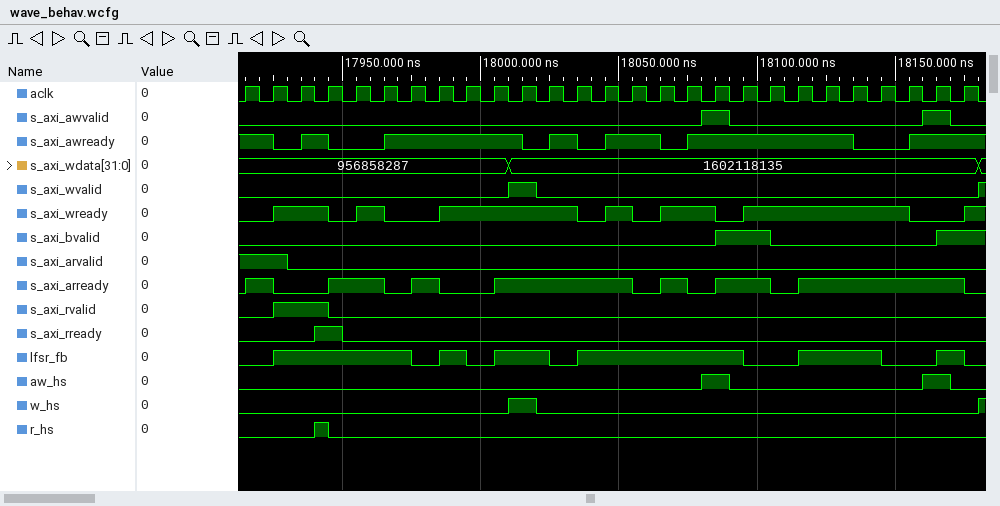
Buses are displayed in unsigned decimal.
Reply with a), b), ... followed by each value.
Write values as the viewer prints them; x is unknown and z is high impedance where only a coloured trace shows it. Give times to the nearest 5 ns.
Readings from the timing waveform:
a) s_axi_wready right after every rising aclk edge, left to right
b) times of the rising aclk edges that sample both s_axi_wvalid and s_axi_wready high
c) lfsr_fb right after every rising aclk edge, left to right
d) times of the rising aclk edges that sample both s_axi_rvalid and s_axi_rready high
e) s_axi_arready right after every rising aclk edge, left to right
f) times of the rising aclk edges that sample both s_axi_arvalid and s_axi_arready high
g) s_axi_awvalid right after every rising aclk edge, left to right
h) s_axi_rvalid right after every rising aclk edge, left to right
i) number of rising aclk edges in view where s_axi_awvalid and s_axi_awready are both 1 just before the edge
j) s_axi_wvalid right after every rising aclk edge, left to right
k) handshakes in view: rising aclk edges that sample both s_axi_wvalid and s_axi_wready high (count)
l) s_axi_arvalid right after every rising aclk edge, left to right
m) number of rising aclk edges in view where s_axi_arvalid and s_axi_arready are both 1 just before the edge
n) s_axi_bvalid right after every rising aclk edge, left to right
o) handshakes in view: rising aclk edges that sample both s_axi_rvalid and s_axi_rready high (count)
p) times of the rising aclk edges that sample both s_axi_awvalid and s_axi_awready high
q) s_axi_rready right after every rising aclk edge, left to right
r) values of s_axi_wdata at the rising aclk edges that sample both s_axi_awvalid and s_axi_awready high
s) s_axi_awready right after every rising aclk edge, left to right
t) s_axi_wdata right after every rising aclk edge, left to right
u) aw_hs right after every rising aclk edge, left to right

a) 0 1 1 0 1 0 0 1 1 1 1 1 0 1 0 1 1 0 1 1 1 1 1 1 0 0 1
b) 18015 ns
c) 0 1 1 1 1 1 0 1 0 1 1 0 1 1 1 1 1 1 0 0 1 1 1 0 0 1 0
d) 17945 ns
e) 1 0 0 1 1 0 1 0 0 1 1 1 1 1 0 1 0 1 1 0 1 1 1 1 1 1 0
f) 17925 ns
g) 0 0 0 0 0 0 0 0 0 0 0 0 0 0 0 0 0 1 0 0 0 0 0 0 0 1 0
h) 0 1 1 0 0 0 0 0 0 0 0 0 0 0 0 0 0 0 0 0 0 0 0 0 0 0 0
i) 2
j) 0 0 0 0 0 0 0 0 0 0 1 0 0 0 0 0 0 0 0 0 0 0 0 0 0 0 0
k) 1
l) 1 1 0 0 0 0 0 0 0 0 0 0 0 0 0 0 0 0 0 0 0 0 0 0 0 0 0
m) 1
n) 0 0 0 0 0 0 0 0 0 0 0 0 0 0 0 0 0 1 1 0 0 0 0 0 0 1 1
o) 1
p) 18085 ns, 18165 ns
q) 0 0 0 1 0 0 0 0 0 0 0 0 0 0 0 0 0 0 0 0 0 0 0 0 0 0 0
r) 1602118135, 1602118135
s) 1 0 1 0 0 1 1 1 1 1 0 1 0 1 1 0 1 1 1 1 1 1 0 0 1 1 1
t) 956858287, 956858287, 956858287, 956858287, 956858287, 956858287, 956858287, 956858287, 956858287, 956858287, 1602118135, 1602118135, 1602118135, 1602118135, 1602118135, 1602118135, 1602118135, 1602118135, 1602118135, 1602118135, 1602118135, 1602118135, 1602118135, 1602118135, 1602118135, 1602118135, 1602118135
u) 0 0 0 0 0 0 0 0 0 0 0 0 0 0 0 0 0 1 0 0 0 0 0 0 0 1 0
